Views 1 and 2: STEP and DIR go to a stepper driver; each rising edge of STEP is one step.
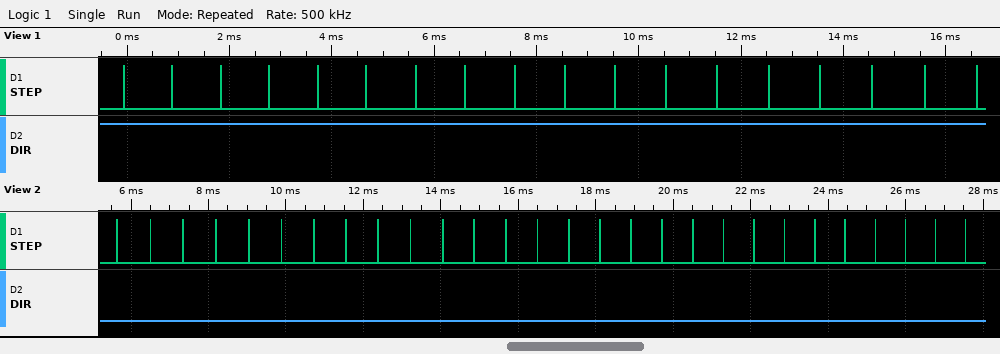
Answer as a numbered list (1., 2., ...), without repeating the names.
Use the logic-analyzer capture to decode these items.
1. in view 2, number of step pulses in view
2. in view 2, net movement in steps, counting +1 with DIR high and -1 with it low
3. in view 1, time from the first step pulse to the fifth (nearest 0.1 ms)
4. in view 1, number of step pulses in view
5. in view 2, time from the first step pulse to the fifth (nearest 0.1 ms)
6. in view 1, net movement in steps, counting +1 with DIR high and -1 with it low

1. 28
2. -28
3. 3.8 ms
4. 18
5. 3.4 ms
6. +18
